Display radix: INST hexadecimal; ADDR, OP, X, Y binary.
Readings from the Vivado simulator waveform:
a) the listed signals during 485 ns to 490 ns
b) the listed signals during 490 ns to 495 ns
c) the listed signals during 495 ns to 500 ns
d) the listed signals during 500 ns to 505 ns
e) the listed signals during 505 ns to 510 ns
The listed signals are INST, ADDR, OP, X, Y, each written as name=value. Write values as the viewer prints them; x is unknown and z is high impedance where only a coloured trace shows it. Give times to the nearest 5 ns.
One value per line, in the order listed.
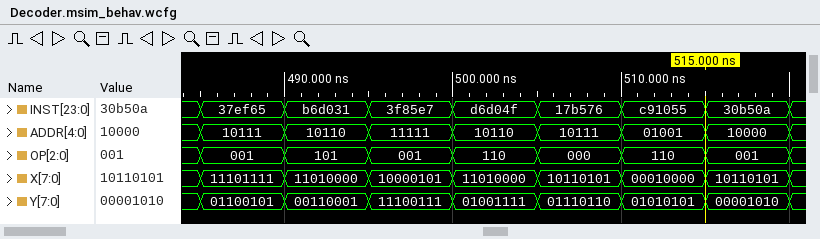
INST=37ef65, ADDR=10111, OP=001, X=11101111, Y=01100101
INST=b6d031, ADDR=10110, OP=101, X=11010000, Y=00110001
INST=3f85e7, ADDR=11111, OP=001, X=10000101, Y=11100111
INST=d6d04f, ADDR=10110, OP=110, X=11010000, Y=01001111
INST=17b576, ADDR=10111, OP=000, X=10110101, Y=01110110
